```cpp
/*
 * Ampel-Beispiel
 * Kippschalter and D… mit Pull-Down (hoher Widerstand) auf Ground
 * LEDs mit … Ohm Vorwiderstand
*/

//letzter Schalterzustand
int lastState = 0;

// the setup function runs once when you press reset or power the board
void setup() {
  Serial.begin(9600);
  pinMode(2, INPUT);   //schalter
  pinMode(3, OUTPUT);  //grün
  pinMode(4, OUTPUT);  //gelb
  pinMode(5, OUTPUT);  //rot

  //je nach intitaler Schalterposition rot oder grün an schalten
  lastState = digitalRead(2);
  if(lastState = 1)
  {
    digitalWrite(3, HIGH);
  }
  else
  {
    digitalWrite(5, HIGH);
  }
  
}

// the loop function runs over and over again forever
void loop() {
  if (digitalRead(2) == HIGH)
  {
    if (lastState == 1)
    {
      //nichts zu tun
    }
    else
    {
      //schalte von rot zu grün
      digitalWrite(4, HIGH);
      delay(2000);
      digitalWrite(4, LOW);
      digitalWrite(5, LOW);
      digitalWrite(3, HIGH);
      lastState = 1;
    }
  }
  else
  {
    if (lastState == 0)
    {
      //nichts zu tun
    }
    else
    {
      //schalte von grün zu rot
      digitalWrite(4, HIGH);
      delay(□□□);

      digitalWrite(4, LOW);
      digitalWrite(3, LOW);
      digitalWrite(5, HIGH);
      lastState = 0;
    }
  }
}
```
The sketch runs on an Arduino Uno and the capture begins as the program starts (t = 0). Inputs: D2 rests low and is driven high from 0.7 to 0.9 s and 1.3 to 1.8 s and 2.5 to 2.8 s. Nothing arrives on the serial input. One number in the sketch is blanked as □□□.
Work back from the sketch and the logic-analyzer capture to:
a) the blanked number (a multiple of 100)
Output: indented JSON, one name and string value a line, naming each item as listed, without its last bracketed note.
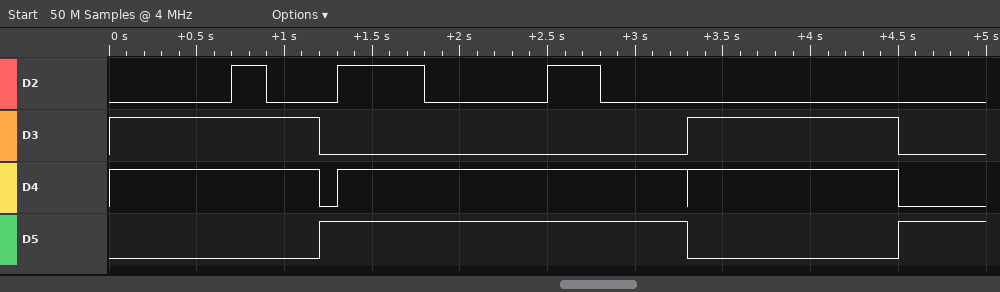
{
  "the blanked number": "1200"
}
